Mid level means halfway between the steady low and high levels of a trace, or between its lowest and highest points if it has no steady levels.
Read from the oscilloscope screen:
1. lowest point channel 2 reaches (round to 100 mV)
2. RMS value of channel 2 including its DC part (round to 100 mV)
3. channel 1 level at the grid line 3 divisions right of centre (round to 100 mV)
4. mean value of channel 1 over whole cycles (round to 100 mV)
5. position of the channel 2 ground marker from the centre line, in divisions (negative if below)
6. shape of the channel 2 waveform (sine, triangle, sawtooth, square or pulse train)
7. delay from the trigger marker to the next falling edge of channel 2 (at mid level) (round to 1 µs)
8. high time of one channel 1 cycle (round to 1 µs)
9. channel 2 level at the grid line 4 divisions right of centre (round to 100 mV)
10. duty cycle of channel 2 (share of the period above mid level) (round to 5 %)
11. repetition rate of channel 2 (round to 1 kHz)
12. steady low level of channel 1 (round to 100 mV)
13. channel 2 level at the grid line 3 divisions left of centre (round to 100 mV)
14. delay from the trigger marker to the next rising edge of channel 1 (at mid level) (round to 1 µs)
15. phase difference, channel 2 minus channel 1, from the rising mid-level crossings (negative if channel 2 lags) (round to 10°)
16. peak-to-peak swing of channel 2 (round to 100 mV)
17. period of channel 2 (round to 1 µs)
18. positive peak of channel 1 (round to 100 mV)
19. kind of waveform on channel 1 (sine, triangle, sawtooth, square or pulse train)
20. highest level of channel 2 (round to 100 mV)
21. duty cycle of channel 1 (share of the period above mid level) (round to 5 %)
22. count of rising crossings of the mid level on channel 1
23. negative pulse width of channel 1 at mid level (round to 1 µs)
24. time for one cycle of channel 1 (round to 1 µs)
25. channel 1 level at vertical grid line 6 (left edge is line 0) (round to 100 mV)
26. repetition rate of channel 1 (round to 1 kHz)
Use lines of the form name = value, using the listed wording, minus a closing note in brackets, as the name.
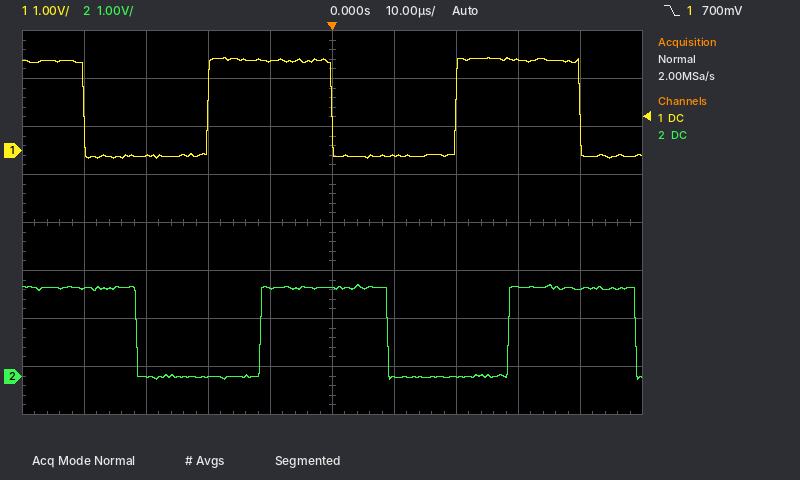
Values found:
lowest point channel 2 reaches = -100 mV
RMS value of channel 2 including its DC part = 1.3 V
channel 1 level at the grid line 3 divisions right of centre = 1.9 V
mean value of channel 1 over whole cycles = 900 mV
position of the channel 2 ground marker from the centre line, in divisions = -3.2 div
shape of the channel 2 waveform = square
delay from the trigger marker to the next falling edge of channel 2 (at mid level) = 9 µs
high time of one channel 1 cycle = 20 µs
channel 2 level at the grid line 4 divisions right of centre = 1.8 V
duty cycle of channel 2 (share of the period above mid level) = 50 %
repetition rate of channel 2 = 25 kHz
steady low level of channel 1 = -100 mV
channel 2 level at the grid line 3 divisions left of centre = 0.0 V
delay from the trigger marker to the next rising edge of channel 1 (at mid level) = 20 µs
phase difference, channel 2 minus channel 1, from the rising mid-level crossings (negative if channel 2 lags) = -80°
peak-to-peak swing of channel 2 = 2.0 V
period of channel 2 = 40 µs
positive peak of channel 1 = 1.9 V
kind of waveform on channel 1 = square
highest level of channel 2 = 1.9 V
duty cycle of channel 1 (share of the period above mid level) = 50 %
count of rising crossings of the mid level on channel 1 = 2
negative pulse width of channel 1 at mid level = 20 µs
time for one cycle of channel 1 = 40 µs
channel 1 level at vertical grid line 6 (left edge is line 0) = -100 mV
repetition rate of channel 1 = 25 kHz
